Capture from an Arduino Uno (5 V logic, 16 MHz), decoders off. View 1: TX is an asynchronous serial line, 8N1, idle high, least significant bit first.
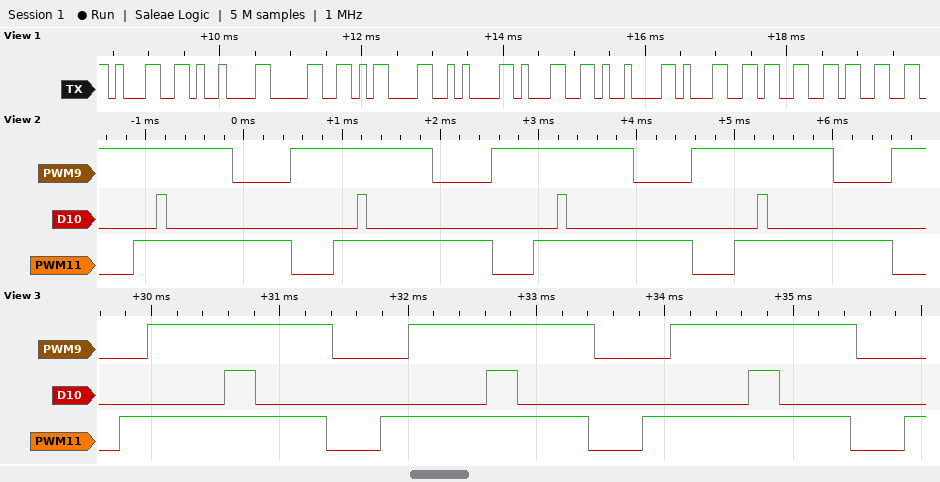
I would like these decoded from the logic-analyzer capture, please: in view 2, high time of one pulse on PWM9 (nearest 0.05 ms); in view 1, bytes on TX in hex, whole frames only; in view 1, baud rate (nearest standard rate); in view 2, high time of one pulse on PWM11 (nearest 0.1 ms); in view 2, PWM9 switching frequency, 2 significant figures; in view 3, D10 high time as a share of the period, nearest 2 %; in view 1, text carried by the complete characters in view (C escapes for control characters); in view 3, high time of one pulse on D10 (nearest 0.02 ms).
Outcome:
1.45 ms
31 09 30 0D 0A 31 09 31 33 33
9600 baud
1.6 ms
490 Hz
12 %
"1\t0\r\n1\t133"
0.24 ms
